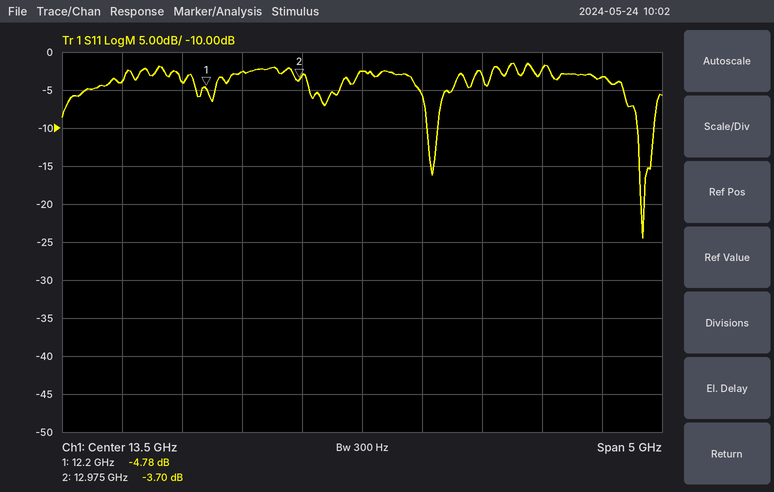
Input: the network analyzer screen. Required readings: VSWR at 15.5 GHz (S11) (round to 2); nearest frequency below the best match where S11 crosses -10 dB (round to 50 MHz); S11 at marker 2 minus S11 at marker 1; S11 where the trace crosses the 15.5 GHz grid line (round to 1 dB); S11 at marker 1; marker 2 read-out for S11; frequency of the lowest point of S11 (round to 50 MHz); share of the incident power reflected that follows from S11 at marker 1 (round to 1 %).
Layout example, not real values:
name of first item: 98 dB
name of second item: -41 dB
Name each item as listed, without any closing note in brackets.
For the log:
VSWR at 15.5 GHz (S11): 6
nearest frequency below the best match where S11 crosses -10 dB: 15.80 GHz
S11 at marker 2 minus S11 at marker 1: 1.08 dB
S11 where the trace crosses the 15.5 GHz grid line: -3 dB
S11 at marker 1: -4.78 dB
marker 2 read-out for S11: -3.70 dB
frequency of the lowest point of S11: 15.85 GHz
share of the incident power reflected that follows from S11 at marker 1: 33 %
